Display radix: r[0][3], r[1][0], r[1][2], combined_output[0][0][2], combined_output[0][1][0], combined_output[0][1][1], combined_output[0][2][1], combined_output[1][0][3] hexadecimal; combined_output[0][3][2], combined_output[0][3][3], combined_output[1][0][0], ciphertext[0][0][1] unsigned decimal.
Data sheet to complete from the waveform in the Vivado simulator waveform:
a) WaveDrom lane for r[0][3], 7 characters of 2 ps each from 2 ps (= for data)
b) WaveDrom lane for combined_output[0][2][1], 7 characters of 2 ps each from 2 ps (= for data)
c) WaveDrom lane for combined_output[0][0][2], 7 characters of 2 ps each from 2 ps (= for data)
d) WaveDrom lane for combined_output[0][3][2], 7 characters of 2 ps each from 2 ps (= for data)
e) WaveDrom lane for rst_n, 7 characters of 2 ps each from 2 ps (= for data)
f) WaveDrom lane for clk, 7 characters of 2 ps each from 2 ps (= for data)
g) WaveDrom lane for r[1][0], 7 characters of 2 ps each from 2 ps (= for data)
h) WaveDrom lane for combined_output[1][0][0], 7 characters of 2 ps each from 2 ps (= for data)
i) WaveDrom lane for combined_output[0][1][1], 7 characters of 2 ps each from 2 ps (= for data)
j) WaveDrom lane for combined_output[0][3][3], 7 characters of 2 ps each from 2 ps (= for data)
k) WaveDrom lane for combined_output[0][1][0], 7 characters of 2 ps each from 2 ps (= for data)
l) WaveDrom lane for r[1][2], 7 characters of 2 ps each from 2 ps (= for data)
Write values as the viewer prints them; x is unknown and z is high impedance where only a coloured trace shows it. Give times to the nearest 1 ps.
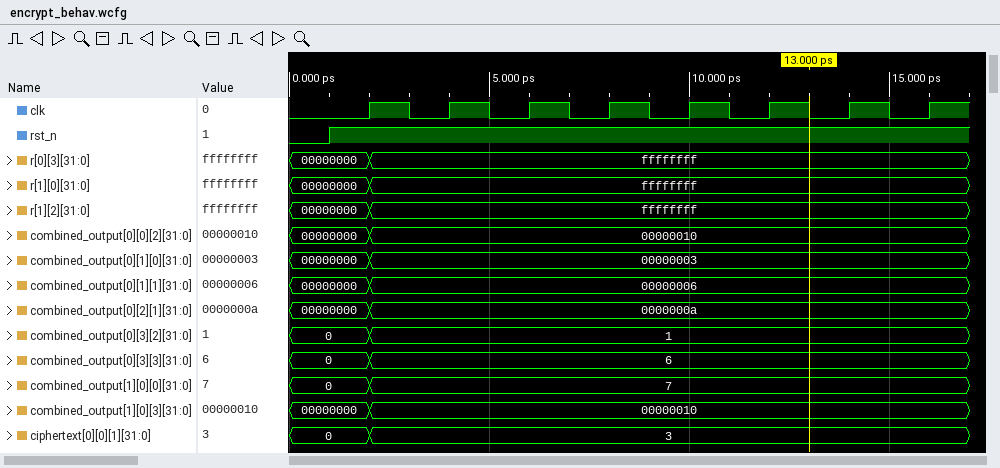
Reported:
{name: 'r[0][3]', wave: '=......', data: 'ffffffff'}
{name: 'combined_output[0][2][1]', wave: '=......', data: '0000000a'}
{name: 'combined_output[0][0][2]', wave: '=......', data: '00000010'}
{name: 'combined_output[0][3][2]', wave: '=......', data: '1'}
{name: 'rst_n', wave: '1......'}
{name: 'clk', wave: 'p......'}
{name: 'r[1][0]', wave: '=......', data: 'ffffffff'}
{name: 'combined_output[1][0][0]', wave: '=......', data: '7'}
{name: 'combined_output[0][1][1]', wave: '=......', data: '00000006'}
{name: 'combined_output[0][3][3]', wave: '=......', data: '6'}
{name: 'combined_output[0][1][0]', wave: '=......', data: '00000003'}
{name: 'r[1][2]', wave: '=......', data: 'ffffffff'}
